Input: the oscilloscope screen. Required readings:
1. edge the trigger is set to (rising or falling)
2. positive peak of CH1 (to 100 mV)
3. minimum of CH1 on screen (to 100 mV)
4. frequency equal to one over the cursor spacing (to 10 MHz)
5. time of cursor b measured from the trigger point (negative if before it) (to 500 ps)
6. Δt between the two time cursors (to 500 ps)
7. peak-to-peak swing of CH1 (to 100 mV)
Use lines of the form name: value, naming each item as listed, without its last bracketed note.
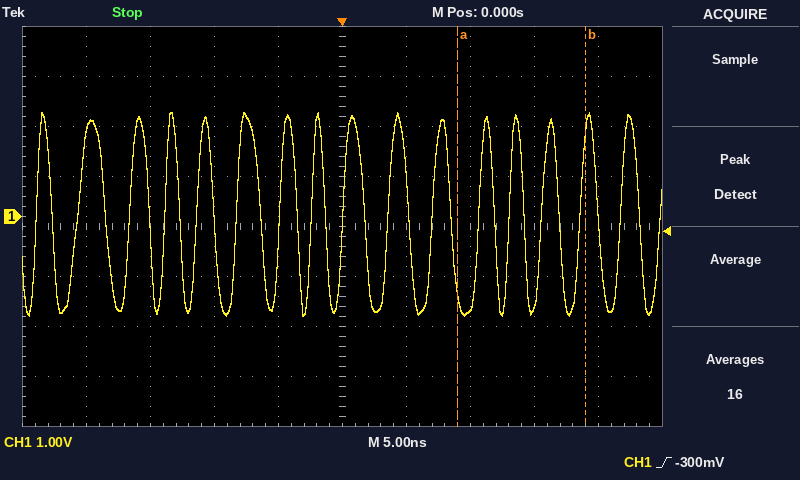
edge the trigger is set to: rising
positive peak of CH1: 2.1 V
minimum of CH1 on screen: -2.0 V
frequency equal to one over the cursor spacing: 100 MHz
time of cursor b measured from the trigger point (negative if before it): +19.0 ns
Δt between the two time cursors: 10.0 ns
peak-to-peak swing of CH1: 4.1 V
